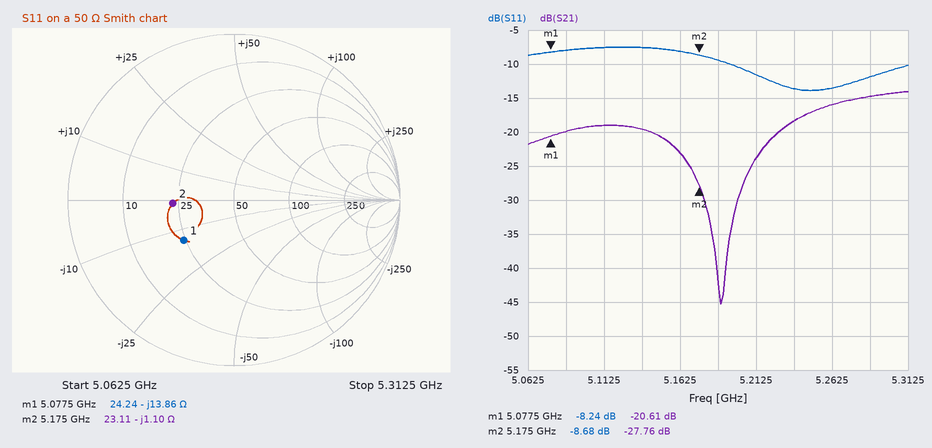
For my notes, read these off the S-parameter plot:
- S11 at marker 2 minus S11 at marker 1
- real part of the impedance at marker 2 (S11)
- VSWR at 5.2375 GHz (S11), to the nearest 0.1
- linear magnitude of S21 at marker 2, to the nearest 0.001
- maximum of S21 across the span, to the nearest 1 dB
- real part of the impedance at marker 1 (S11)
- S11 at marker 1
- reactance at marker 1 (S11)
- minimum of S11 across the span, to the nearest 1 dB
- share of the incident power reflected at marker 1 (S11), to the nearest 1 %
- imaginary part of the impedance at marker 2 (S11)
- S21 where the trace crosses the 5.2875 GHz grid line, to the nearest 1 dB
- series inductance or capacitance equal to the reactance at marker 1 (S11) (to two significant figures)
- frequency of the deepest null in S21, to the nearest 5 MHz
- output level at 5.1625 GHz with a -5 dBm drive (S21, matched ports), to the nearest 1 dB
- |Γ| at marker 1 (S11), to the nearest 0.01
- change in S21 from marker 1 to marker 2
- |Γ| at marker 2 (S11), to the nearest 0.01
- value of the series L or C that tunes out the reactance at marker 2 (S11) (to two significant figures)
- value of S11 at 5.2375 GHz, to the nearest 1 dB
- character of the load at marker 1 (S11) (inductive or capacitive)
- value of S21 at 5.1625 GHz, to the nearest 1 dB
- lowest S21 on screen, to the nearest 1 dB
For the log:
-0.44 dB
23.11 Ω
1.5
0.041
-14 dB
24.24 Ω
-8.24 dB
-13.86 Ω
-14 dB
15 %
-1.10 Ω
-15 dB
2.3 pF
5.190 GHz
-28 dBm
0.39
-7.15 dB
0.37
34 pH
-14 dB
capacitive
-23 dB
-45 dB
